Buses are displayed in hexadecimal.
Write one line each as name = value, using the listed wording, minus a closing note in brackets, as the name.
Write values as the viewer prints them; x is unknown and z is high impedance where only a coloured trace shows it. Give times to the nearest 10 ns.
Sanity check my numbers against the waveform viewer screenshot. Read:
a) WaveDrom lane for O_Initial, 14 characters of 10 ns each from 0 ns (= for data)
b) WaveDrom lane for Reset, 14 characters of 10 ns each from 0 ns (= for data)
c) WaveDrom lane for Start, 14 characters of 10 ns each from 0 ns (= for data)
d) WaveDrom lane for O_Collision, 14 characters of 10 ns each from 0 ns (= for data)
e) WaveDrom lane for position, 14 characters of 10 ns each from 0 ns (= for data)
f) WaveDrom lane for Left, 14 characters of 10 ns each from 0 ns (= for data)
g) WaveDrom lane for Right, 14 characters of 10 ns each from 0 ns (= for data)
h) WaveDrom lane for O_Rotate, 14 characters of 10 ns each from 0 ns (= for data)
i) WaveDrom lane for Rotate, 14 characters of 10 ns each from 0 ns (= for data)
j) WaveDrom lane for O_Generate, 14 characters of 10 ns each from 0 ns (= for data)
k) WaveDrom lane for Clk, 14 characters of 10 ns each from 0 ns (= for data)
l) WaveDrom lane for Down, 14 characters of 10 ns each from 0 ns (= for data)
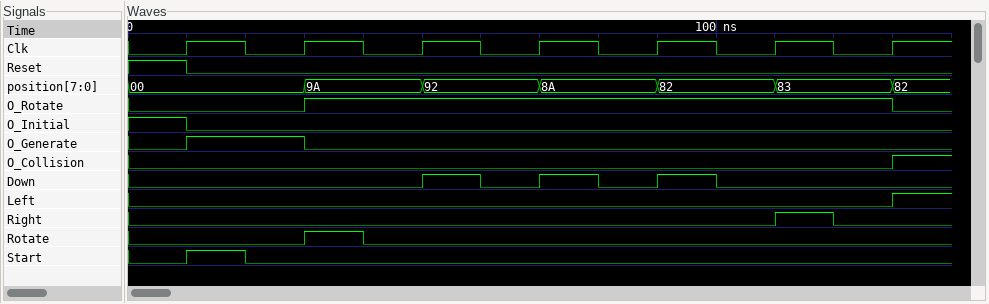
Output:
WaveDrom lane for O_Initial, 14 characters of 10 ns each from 0 ns = {name: 'O_Initial', wave: '10............'}
WaveDrom lane for Reset, 14 characters of 10 ns each from 0 ns = {name: 'Reset', wave: '10............'}
WaveDrom lane for Start, 14 characters of 10 ns each from 0 ns = {name: 'Start', wave: '010...........'}
WaveDrom lane for O_Collision, 14 characters of 10 ns each from 0 ns = {name: 'O_Collision', wave: '0............1'}
WaveDrom lane for position, 14 characters of 10 ns each from 0 ns = {name: 'position', wave: '=..=.=.=.=.=.=', data: '00 9A 92 8A 82 83 82'}
WaveDrom lane for Left, 14 characters of 10 ns each from 0 ns = {name: 'Left', wave: '0............1'}
WaveDrom lane for Right, 14 characters of 10 ns each from 0 ns = {name: 'Right', wave: '0..........10.'}
WaveDrom lane for O_Rotate, 14 characters of 10 ns each from 0 ns = {name: 'O_Rotate', wave: '0..1.........0'}
WaveDrom lane for Rotate, 14 characters of 10 ns each from 0 ns = {name: 'Rotate', wave: '0..10.........'}
WaveDrom lane for O_Generate, 14 characters of 10 ns each from 0 ns = {name: 'O_Generate', wave: '01.0..........'}
WaveDrom lane for Clk, 14 characters of 10 ns each from 0 ns = {name: 'Clk', wave: '01010101010101'}
WaveDrom lane for Down, 14 characters of 10 ns each from 0 ns = {name: 'Down', wave: '0....101010...'}
